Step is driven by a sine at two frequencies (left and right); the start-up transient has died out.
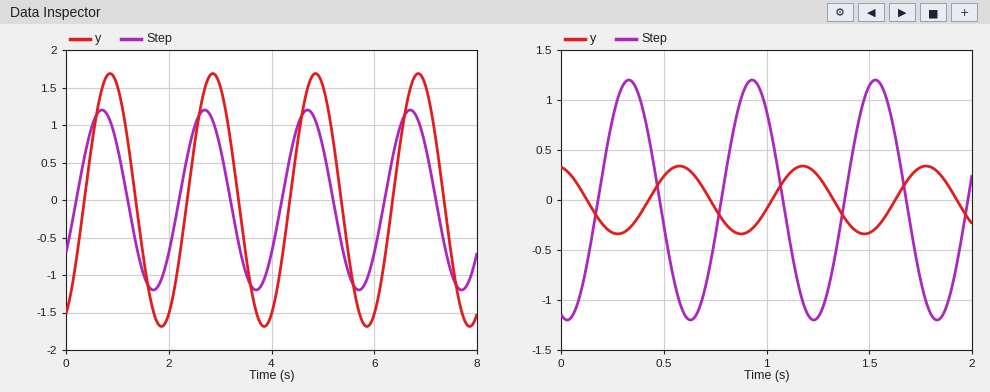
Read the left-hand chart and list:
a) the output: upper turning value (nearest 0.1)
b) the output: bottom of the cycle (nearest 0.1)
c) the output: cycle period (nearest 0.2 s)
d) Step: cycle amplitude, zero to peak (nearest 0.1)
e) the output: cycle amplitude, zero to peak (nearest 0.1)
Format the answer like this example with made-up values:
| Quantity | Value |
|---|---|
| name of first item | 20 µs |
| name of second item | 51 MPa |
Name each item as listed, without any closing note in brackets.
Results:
| Quantity | Value |
|---|---|
| the output: upper turning value | 1.7 |
| the output: bottom of the cycle | -1.7 |
| the output: cycle period | 2.0 s |
| Step: cycle amplitude, zero to peak | 1.2 |
| the output: cycle amplitude, zero to peak | 1.7 |
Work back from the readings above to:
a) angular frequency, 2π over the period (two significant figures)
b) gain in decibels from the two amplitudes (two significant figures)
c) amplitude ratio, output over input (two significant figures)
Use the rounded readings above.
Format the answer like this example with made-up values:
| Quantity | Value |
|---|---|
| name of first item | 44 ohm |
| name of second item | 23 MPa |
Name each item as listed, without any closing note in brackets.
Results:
| Quantity | Value |
|---|---|
| angular frequency, 2π over the period | 3.1 rad/s |
| gain in decibels from the two amplitudes | 3.0 dB |
| amplitude ratio, output over input | 1.4 |
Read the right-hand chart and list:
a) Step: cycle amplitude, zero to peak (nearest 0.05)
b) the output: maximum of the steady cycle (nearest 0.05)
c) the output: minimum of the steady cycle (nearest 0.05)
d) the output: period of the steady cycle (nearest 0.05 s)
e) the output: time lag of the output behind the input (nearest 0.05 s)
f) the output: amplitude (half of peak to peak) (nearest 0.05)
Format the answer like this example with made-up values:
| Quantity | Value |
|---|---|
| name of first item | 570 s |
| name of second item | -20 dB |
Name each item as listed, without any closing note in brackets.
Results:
| Quantity | Value |
|---|---|
| Step: cycle amplitude, zero to peak | 1.20 |
| the output: maximum of the steady cycle | 0.35 |
| the output: minimum of the steady cycle | -0.35 |
| the output: period of the steady cycle | 0.60 s |
| the output: time lag of the output behind the input | 0.25 s |
| the output: amplitude (half of peak to peak) | 0.35 |
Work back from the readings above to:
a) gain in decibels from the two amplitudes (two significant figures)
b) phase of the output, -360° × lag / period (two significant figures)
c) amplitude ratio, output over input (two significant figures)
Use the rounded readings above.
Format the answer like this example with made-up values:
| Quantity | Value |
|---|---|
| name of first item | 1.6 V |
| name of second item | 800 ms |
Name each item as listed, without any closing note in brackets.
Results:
| Quantity | Value |
|---|---|
| gain in decibels from the two amplitudes | -11 dB |
| phase of the output, -360° × lag / period | -150° |
| amplitude ratio, output over input | 0.29 |
